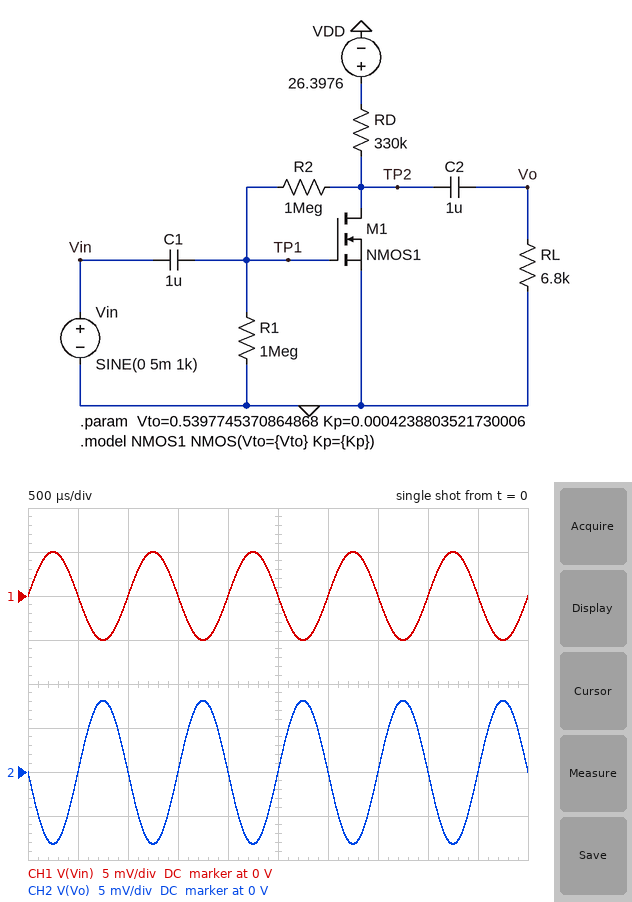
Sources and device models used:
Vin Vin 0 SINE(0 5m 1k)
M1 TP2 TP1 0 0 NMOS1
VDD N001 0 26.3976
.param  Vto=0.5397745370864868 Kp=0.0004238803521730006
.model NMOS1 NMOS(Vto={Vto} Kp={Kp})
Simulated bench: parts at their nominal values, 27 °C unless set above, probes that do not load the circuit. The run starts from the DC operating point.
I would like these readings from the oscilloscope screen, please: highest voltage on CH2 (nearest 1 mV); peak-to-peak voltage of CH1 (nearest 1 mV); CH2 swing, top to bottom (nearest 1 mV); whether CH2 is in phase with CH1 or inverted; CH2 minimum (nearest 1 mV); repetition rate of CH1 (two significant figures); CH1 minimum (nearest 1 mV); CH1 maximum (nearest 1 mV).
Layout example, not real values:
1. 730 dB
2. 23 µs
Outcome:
1. 8 mV
2. 10 mV
3. 16 mV
4. inverted
5. -8 mV
6. 1.0 kHz
7. -5 mV
8. 5 mV
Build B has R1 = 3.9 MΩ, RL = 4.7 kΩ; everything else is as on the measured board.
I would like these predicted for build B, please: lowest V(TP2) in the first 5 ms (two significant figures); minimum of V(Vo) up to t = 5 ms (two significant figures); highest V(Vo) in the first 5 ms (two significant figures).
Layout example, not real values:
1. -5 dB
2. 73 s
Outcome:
1. 1.4 V
2. -5.8 mV
3. 5.8 mV
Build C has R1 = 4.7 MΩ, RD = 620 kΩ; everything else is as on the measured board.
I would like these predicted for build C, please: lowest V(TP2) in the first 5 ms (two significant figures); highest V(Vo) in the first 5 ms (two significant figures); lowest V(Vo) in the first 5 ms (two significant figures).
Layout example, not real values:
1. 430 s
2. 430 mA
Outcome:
1. 1.2 V
2. 6.1 mV
3. -6.2 mV
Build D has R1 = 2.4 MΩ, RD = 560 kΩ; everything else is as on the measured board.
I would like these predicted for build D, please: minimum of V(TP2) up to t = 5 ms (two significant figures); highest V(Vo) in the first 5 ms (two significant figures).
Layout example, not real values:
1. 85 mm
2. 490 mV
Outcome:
1. 1.4 V
2. 6.4 mV
